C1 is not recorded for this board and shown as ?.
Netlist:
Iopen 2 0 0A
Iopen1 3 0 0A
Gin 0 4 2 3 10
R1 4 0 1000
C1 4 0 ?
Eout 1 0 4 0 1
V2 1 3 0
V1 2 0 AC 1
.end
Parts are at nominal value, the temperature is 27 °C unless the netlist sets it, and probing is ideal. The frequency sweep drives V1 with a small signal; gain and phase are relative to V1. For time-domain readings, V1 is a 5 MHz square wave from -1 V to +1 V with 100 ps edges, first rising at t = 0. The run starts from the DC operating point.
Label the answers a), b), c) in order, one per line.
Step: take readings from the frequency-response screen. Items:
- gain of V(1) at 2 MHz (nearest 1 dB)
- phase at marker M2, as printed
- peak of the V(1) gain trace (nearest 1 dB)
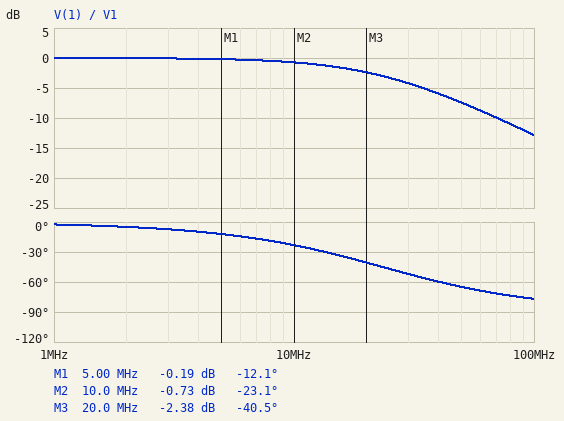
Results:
a) 0 dB
b) -23.1 deg
c) 0 dB
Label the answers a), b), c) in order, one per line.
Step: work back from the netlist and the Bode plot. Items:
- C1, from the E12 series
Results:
a) 68 nF
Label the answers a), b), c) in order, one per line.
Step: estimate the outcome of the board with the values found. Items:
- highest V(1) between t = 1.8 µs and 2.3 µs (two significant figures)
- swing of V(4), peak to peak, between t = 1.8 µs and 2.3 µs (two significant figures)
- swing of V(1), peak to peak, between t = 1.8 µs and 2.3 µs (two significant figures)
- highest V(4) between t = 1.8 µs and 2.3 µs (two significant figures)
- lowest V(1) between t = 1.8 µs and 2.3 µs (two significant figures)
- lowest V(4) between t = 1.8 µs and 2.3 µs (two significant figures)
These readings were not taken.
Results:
a) 1.0 V
b) 2.0 V
c) 2.0 V
d) 1.0 V
e) -1.0 V
f) -1.0 V
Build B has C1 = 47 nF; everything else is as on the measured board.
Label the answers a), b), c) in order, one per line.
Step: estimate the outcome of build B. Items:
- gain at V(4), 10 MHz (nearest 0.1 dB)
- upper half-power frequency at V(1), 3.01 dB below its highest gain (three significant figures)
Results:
a) -0.4 dB
b) 33.9 MHz
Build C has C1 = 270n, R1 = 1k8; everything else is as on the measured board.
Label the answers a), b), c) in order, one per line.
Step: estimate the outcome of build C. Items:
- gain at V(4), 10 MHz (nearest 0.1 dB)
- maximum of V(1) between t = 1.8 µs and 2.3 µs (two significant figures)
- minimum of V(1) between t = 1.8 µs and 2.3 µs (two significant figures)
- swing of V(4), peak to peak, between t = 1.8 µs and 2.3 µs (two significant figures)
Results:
a) -5.9 dB
b) 950 mV
c) -950 mV
d) 1.9 V
